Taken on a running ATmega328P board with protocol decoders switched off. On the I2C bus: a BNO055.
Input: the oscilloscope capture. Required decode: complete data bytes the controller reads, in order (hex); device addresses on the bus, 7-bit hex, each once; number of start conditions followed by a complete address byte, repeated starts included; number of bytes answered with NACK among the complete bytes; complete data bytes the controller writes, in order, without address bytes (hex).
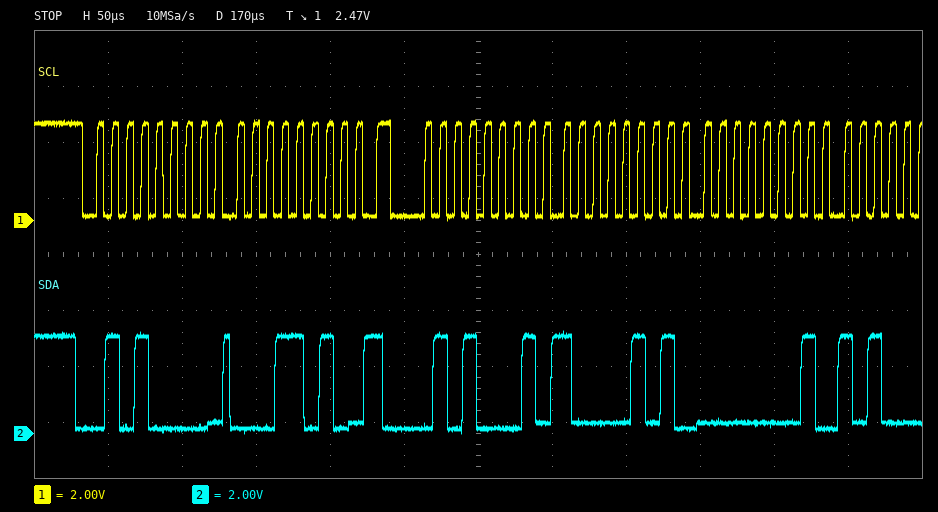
85 01
0x28
2
0
1A
